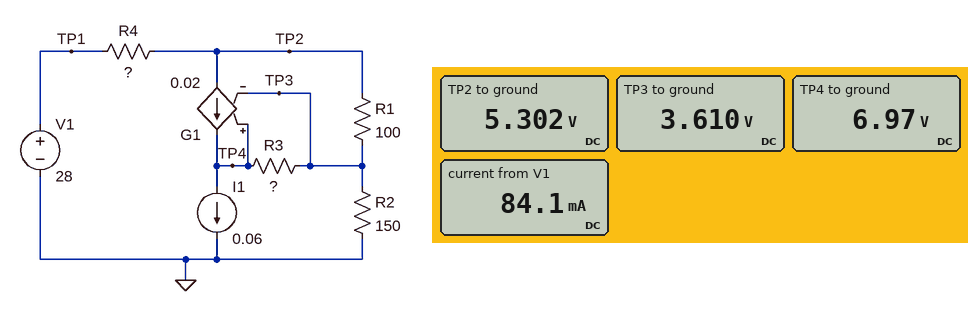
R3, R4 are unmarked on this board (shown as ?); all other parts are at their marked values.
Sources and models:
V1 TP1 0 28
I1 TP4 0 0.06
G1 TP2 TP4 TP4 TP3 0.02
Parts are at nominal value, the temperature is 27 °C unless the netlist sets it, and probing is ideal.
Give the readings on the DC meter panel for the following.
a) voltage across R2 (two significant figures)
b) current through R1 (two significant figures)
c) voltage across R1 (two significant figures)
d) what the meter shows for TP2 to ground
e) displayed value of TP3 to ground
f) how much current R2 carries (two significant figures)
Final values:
3.6 V
17 mA
1.7 V
5.302 V
3.610 V
24 mA
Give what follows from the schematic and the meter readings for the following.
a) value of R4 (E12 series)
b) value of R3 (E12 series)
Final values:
270 Ω
470 Ω
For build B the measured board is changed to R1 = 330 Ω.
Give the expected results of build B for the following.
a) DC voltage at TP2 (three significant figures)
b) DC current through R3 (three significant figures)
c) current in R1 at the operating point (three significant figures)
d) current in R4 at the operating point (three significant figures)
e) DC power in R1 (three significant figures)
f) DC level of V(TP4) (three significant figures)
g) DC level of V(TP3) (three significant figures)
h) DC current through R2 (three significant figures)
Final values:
6.70 V
7.14 mA
11.7 mA
78.9 mA
45.4 mW
6.19 V
2.83 V
18.9 mA
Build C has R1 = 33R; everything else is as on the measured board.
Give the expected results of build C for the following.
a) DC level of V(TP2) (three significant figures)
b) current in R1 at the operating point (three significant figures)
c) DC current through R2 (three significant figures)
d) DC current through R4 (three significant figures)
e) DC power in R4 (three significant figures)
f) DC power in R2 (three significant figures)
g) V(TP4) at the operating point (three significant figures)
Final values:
4.63 V
19.4 mA
26.6 mA
86.6 mA
2.02 W
106 mW
7.34 V
